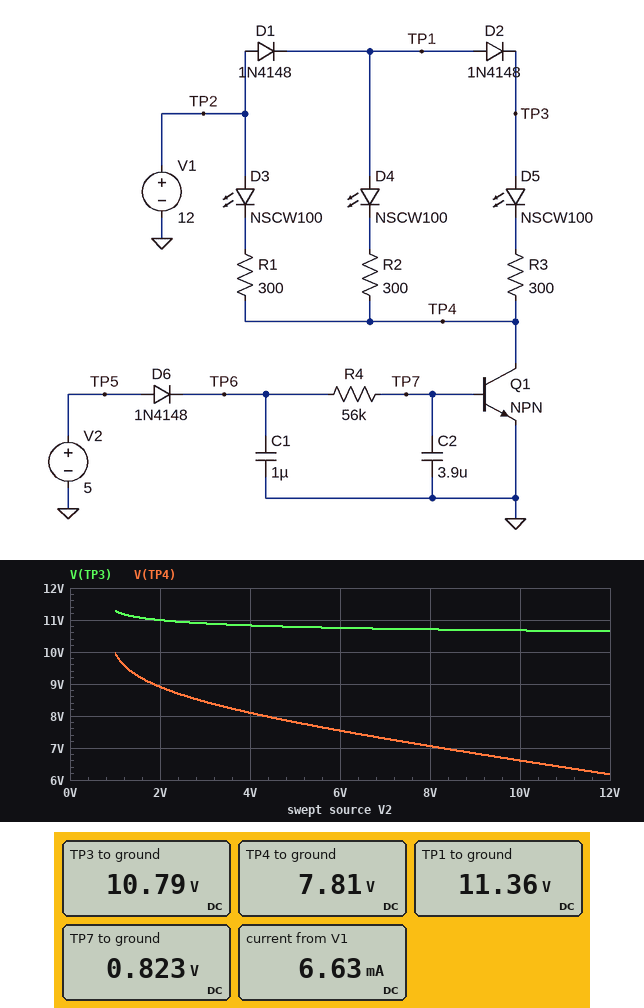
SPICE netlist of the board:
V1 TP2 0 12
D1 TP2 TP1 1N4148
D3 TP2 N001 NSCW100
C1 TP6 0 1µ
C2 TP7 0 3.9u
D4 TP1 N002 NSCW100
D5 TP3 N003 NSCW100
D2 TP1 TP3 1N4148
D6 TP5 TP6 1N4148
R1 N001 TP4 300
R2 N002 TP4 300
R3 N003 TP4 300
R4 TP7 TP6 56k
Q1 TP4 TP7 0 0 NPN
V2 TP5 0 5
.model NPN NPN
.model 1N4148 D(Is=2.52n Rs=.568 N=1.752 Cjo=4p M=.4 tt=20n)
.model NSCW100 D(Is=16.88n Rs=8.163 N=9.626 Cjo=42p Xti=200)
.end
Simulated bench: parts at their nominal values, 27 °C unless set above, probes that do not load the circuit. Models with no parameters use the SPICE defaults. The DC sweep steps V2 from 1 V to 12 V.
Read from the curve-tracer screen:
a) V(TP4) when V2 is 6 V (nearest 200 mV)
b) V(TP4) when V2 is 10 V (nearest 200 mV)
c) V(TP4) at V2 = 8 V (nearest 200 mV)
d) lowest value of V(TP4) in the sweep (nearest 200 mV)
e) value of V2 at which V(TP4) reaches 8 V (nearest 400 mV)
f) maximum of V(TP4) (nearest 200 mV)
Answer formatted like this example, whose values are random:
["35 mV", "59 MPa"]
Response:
["7.6 V", "6.6 V", "7.0 V", "6.2 V", "4.4 V", "10.0 V"]
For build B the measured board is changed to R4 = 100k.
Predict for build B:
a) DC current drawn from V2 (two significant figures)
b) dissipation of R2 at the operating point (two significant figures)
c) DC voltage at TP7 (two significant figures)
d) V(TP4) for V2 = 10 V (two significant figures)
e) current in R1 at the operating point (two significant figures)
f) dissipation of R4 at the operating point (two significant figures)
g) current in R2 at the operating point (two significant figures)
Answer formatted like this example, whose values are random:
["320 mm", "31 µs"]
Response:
["38 µA", "340 µW", "810 mV", "7.5 V", "2.4 mA", "140 µW", "1.1 mA"]
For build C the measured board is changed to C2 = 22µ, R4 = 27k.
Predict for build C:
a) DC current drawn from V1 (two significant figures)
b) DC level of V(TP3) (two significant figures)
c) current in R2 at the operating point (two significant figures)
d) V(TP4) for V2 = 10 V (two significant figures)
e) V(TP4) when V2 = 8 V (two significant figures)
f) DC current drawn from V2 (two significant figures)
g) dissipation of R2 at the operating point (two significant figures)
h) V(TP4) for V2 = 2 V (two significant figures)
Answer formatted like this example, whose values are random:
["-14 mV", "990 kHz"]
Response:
["14 mA", "11 V", "4.4 mA", "4.7 V", "5.5 V", "140 µA", "5.9 mW", "8.5 V"]
